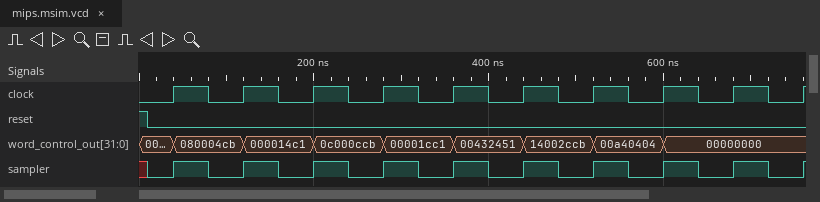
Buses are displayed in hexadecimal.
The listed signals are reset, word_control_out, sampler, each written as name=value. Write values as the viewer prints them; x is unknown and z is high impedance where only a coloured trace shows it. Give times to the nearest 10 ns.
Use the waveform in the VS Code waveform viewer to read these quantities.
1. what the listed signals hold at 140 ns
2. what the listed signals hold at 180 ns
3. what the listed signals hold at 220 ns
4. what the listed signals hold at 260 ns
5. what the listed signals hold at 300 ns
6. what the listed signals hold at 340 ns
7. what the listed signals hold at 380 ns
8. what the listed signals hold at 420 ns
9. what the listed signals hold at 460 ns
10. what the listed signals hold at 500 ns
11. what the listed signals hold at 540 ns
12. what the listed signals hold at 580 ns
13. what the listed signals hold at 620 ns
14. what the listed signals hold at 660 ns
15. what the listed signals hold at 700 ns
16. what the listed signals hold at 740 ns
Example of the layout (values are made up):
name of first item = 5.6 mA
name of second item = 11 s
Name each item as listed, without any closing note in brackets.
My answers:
what the listed signals hold at 140 ns = reset=0, word_control_out=000014c1, sampler=1
what the listed signals hold at 180 ns = reset=0, word_control_out=000014c1, sampler=0
what the listed signals hold at 220 ns = reset=0, word_control_out=0c000ccb, sampler=1
what the listed signals hold at 260 ns = reset=0, word_control_out=0c000ccb, sampler=0
what the listed signals hold at 300 ns = reset=0, word_control_out=00001cc1, sampler=1
what the listed signals hold at 340 ns = reset=0, word_control_out=00001cc1, sampler=0
what the listed signals hold at 380 ns = reset=0, word_control_out=00432451, sampler=1
what the listed signals hold at 420 ns = reset=0, word_control_out=00432451, sampler=0
what the listed signals hold at 460 ns = reset=0, word_control_out=14002ccb, sampler=1
what the listed signals hold at 500 ns = reset=0, word_control_out=14002ccb, sampler=0
what the listed signals hold at 540 ns = reset=0, word_control_out=00a40404, sampler=1
what the listed signals hold at 580 ns = reset=0, word_control_out=00a40404, sampler=0
what the listed signals hold at 620 ns = reset=0, word_control_out=00000000, sampler=1
what the listed signals hold at 660 ns = reset=0, word_control_out=00000000, sampler=0
what the listed signals hold at 700 ns = reset=0, word_control_out=00000000, sampler=1
what the listed signals hold at 740 ns = reset=0, word_control_out=00000000, sampler=0
